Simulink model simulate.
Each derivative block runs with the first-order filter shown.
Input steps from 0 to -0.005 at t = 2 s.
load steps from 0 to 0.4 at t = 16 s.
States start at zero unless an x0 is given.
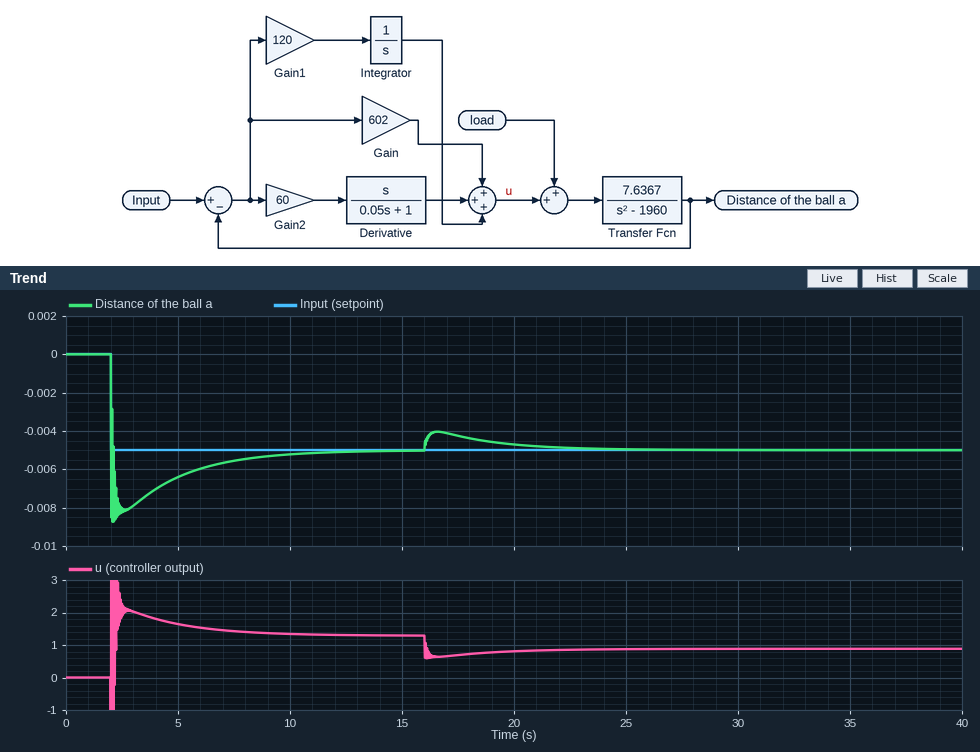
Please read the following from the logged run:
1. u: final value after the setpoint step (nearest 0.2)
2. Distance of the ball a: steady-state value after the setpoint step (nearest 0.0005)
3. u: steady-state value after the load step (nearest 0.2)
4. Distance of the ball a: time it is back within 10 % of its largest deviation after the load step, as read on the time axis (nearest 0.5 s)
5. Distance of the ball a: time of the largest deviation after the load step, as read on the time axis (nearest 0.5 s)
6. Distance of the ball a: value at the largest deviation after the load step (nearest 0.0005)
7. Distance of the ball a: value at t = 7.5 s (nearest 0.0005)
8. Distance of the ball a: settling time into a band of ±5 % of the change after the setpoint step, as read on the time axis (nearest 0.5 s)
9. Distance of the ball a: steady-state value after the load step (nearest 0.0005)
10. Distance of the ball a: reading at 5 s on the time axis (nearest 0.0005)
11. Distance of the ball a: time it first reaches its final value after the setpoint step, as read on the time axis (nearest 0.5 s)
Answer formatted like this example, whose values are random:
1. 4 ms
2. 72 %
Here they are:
1. 1.2
2. -0.0050
3. 0.8
4. 23.0 s
5. 16.5 s
6. -0.0040
7. -0.0055
8. 9.5 s
9. -0.0050
10. -0.0065
11. 2.0 s
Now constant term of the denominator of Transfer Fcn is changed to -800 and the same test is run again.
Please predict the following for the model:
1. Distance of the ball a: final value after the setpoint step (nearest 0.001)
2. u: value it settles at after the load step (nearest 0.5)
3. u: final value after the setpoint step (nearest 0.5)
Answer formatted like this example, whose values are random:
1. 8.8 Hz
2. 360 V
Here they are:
1. -0.005
2. 0.0
3. 0.5
